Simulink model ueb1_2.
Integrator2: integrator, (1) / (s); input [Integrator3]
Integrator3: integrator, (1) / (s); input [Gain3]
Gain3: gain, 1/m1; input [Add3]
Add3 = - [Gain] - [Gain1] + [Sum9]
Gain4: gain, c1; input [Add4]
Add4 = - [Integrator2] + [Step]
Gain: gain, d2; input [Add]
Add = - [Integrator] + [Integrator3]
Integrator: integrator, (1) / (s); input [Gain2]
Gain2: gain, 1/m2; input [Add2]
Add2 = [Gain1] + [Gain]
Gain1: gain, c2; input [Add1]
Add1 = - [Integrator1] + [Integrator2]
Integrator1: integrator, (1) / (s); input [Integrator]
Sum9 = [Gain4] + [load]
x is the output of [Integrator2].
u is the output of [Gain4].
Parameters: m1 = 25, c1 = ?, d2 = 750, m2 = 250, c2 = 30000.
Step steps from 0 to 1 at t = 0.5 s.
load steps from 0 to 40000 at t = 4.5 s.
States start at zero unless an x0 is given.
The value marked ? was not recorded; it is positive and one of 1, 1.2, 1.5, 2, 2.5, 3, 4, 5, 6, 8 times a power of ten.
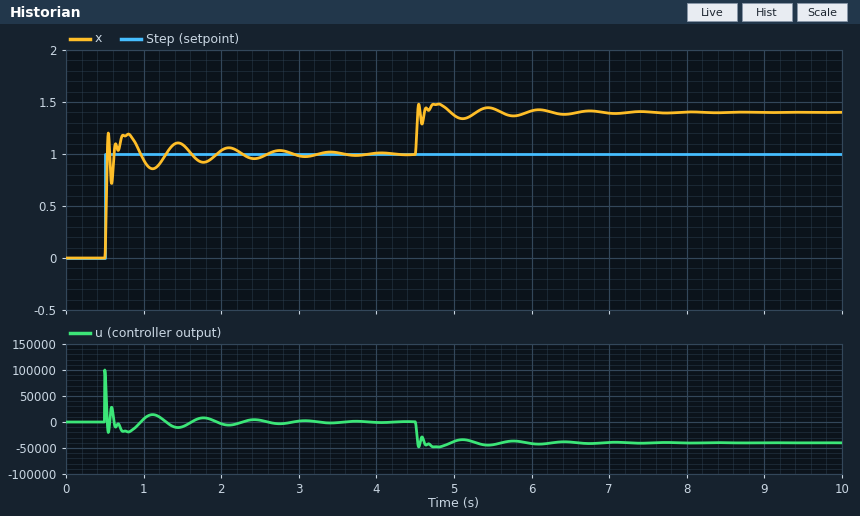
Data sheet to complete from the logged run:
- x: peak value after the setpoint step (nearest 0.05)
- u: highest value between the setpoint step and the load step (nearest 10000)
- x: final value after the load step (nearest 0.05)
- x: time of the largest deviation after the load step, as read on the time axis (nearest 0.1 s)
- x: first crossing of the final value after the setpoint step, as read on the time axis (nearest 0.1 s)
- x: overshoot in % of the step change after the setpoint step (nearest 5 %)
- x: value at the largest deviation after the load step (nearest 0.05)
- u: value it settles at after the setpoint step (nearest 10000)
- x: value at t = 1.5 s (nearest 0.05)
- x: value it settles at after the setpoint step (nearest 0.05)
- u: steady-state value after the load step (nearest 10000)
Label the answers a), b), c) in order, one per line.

a) 1.20
b) 100000
c) 1.40
d) 4.8 s
e) 0.5 s
f) 20 %
g) 1.50
h) 0
i) 1.10
j) 1.00
k) -40000
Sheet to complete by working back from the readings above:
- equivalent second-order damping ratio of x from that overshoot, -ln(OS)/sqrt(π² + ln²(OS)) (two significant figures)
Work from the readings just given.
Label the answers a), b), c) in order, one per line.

a) 0.46
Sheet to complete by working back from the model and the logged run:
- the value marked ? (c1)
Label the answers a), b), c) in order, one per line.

a) 100000
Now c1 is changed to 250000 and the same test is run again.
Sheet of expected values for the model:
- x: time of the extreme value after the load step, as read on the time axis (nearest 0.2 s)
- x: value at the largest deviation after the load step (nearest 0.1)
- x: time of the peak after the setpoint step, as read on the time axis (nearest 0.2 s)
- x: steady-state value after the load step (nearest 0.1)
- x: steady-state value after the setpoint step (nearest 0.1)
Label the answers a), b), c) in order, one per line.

a) 4.6 s
b) 1.2
c) 0.6 s
d) 1.2
e) 1.0
